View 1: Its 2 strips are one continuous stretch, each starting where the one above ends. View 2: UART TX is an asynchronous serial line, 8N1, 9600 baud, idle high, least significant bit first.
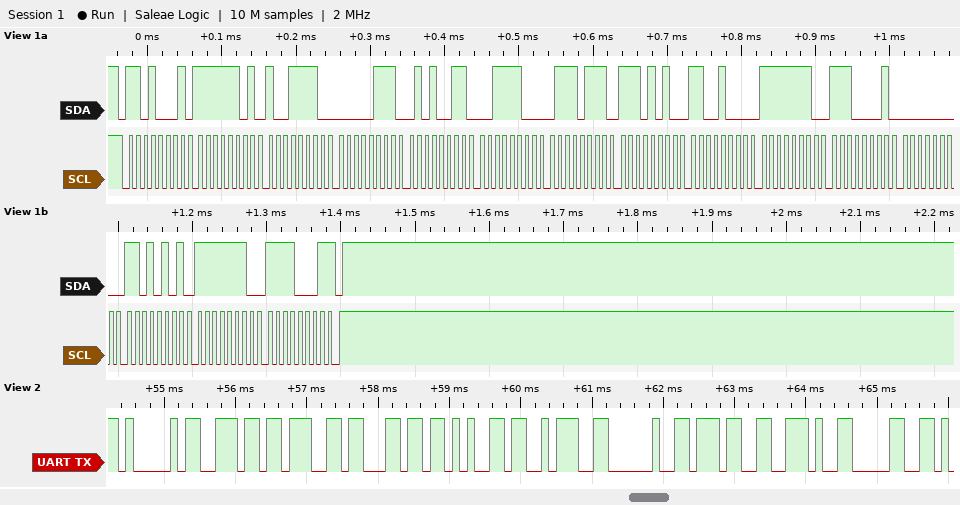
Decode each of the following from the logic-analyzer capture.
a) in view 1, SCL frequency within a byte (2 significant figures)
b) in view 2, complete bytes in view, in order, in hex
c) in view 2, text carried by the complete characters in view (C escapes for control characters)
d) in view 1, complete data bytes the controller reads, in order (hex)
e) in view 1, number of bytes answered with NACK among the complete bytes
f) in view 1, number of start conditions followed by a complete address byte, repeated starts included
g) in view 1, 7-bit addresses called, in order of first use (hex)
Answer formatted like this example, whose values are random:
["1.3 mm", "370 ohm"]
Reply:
["100 kHz", "41 6E 67 6C 65 3A 20 37 2E 30", "\"Angle: 7.0\"", "FD 9E 07 53 3C 77 EA C8 FE E1 00 D5 FE F1", "1", "1", "0x68"]
